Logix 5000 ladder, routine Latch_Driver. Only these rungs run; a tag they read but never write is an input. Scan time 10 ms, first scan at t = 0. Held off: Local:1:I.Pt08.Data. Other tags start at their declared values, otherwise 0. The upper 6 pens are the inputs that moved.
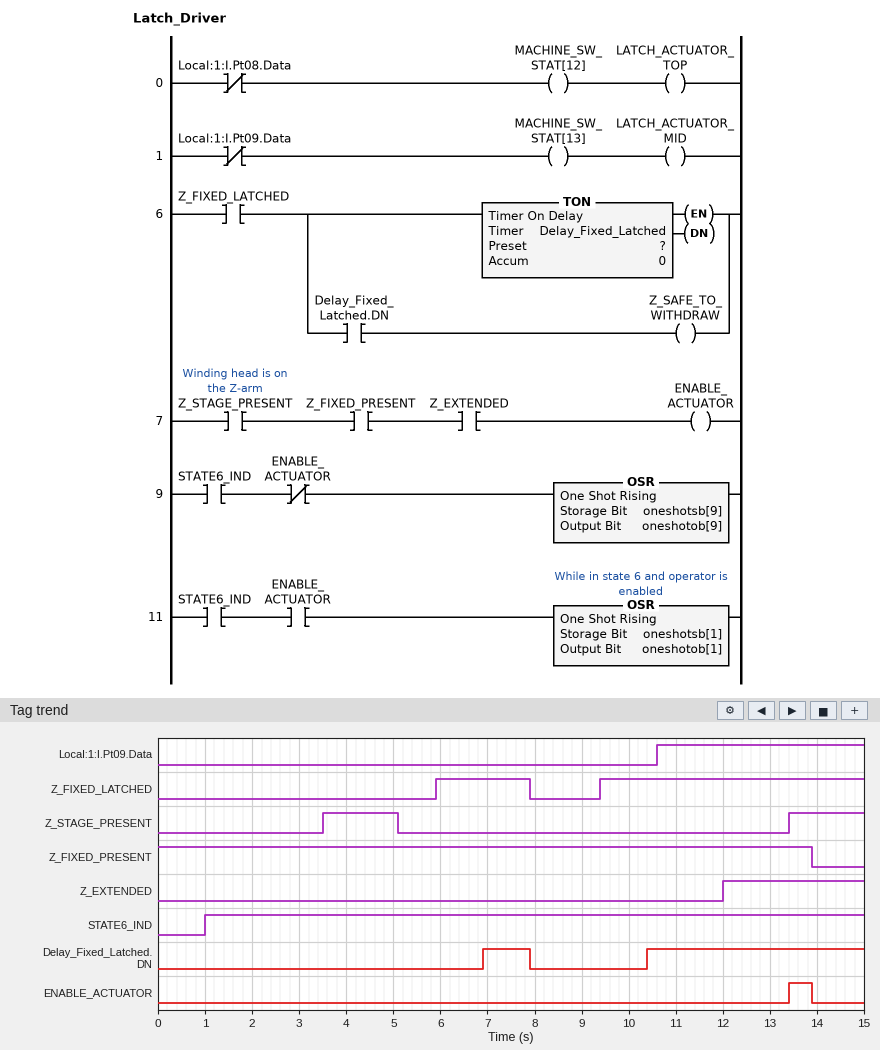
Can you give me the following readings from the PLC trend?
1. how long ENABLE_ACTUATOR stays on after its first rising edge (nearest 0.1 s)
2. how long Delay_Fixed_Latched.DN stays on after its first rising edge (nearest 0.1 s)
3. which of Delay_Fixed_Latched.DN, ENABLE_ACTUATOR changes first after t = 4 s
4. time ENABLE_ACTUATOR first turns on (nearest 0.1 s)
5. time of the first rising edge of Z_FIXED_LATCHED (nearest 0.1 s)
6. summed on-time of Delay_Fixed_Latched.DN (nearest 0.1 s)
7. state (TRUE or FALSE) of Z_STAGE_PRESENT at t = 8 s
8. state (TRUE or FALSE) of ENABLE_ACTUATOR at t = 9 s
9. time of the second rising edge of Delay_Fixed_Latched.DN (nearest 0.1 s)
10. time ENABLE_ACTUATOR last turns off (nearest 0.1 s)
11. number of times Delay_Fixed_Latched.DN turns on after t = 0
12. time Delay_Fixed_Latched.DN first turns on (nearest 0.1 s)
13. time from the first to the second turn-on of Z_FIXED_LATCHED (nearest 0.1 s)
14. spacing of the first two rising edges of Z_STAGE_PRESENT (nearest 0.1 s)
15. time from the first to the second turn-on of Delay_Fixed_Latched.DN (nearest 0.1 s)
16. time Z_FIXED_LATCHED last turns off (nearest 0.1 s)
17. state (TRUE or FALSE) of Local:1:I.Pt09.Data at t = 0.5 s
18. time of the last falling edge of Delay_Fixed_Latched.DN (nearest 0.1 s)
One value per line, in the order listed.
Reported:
0.5 s
1.0 s
Delay_Fixed_Latched.DN
13.4 s
5.9 s
5.6 s
FALSE
FALSE
10.4 s
13.9 s
2
6.9 s
3.5 s
9.9 s
3.5 s
7.9 s
FALSE
7.9 s
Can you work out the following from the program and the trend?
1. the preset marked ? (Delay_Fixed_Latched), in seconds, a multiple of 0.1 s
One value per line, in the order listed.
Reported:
1.0 s
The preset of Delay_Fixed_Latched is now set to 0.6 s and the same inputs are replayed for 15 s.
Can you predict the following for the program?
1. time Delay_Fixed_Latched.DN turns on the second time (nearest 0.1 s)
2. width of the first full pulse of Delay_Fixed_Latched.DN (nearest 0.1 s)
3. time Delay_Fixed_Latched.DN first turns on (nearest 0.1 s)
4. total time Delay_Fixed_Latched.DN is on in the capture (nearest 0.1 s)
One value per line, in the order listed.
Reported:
10.0 s
1.4 s
6.5 s
6.4 s
